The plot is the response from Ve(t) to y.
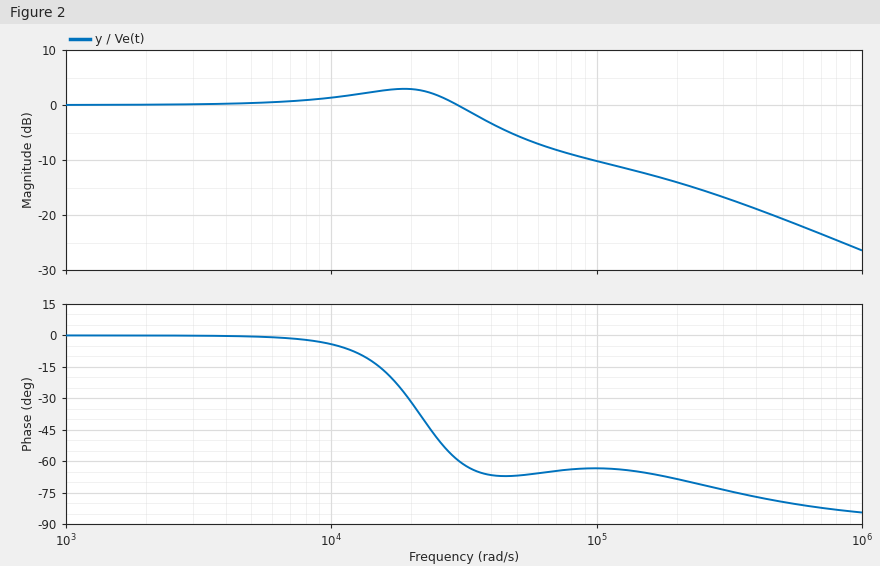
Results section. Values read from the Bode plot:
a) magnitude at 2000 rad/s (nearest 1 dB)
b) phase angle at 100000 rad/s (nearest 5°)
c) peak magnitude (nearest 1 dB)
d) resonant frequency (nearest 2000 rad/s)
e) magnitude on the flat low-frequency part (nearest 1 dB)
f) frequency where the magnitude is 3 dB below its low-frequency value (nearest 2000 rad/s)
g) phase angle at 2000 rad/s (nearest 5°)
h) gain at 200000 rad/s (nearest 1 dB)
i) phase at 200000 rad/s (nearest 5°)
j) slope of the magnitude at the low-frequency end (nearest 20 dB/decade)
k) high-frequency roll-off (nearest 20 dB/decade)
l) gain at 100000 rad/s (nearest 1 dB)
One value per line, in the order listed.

0 dB
-65°
3 dB
18000 rad/s
0 dB
38000 rad/s
0°
-14 dB
-70°
0 dB/decade
-20 dB/decade
-10 dB
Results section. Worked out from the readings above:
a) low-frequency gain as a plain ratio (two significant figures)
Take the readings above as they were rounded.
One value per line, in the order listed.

1.0
